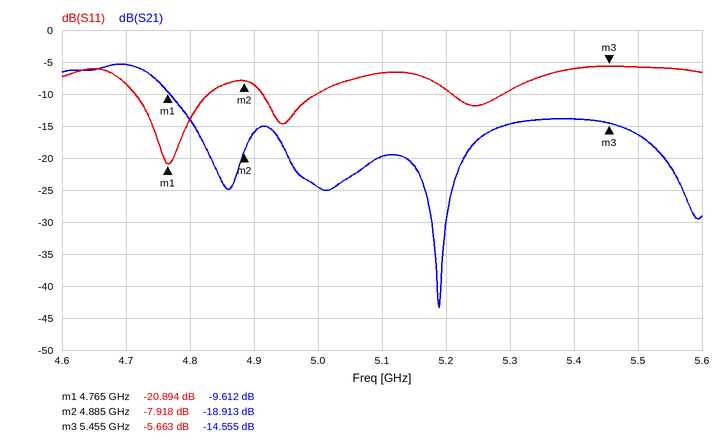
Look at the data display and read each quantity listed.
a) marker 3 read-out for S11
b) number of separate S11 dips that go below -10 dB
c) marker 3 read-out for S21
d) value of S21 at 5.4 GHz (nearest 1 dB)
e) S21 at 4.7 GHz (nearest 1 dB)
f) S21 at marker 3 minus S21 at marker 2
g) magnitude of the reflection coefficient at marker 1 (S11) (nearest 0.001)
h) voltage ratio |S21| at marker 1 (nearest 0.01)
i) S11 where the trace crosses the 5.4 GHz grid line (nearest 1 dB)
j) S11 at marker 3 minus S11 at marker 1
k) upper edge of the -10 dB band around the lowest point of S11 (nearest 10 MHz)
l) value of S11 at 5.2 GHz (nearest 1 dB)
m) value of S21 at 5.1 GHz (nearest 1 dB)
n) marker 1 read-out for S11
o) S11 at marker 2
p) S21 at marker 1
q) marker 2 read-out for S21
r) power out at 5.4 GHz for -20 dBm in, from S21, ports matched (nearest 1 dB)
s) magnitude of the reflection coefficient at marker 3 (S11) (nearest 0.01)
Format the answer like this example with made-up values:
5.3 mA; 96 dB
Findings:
-5.663 dB; 3; -14.555 dB; -14 dB; -5 dB; 4.358 dB; 0.090; 0.33; -6 dB; 15.231 dB; 4.83 GHz; -9 dB; -20 dB; -20.894 dB; -7.918 dB; -9.612 dB; -18.913 dB; -34 dBm; 0.52
